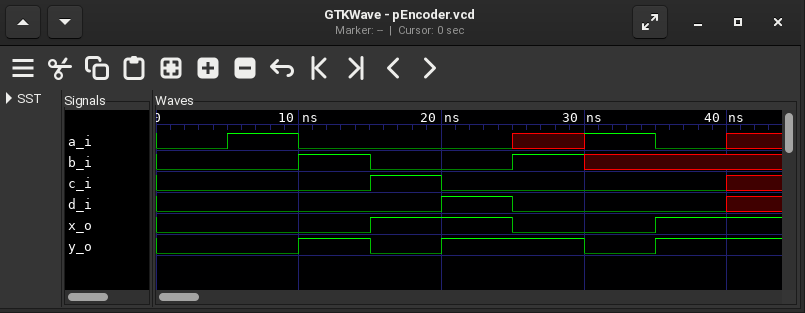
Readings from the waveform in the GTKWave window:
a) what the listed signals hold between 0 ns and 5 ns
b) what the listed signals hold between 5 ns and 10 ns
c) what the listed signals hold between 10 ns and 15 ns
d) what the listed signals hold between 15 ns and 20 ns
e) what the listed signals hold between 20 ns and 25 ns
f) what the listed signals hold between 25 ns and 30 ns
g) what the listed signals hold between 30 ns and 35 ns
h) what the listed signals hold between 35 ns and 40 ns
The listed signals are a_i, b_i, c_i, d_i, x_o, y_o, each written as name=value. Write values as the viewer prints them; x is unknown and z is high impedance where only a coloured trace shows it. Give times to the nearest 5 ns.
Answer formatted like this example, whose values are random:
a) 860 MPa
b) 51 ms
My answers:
a) a_i=0, b_i=0, c_i=0, d_i=0, x_o=0, y_o=0
b) a_i=1, b_i=0, c_i=0, d_i=0, x_o=0, y_o=0
c) a_i=0, b_i=1, c_i=0, d_i=0, x_o=0, y_o=1
d) a_i=0, b_i=0, c_i=1, d_i=0, x_o=1, y_o=0
e) a_i=0, b_i=0, c_i=0, d_i=1, x_o=1, y_o=1
f) a_i=x, b_i=1, c_i=0, d_i=0, x_o=0, y_o=1
g) a_i=1, b_i=x, c_i=0, d_i=0, x_o=0, y_o=0
h) a_i=0, b_i=x, c_i=0, d_i=0, x_o=1, y_o=1
